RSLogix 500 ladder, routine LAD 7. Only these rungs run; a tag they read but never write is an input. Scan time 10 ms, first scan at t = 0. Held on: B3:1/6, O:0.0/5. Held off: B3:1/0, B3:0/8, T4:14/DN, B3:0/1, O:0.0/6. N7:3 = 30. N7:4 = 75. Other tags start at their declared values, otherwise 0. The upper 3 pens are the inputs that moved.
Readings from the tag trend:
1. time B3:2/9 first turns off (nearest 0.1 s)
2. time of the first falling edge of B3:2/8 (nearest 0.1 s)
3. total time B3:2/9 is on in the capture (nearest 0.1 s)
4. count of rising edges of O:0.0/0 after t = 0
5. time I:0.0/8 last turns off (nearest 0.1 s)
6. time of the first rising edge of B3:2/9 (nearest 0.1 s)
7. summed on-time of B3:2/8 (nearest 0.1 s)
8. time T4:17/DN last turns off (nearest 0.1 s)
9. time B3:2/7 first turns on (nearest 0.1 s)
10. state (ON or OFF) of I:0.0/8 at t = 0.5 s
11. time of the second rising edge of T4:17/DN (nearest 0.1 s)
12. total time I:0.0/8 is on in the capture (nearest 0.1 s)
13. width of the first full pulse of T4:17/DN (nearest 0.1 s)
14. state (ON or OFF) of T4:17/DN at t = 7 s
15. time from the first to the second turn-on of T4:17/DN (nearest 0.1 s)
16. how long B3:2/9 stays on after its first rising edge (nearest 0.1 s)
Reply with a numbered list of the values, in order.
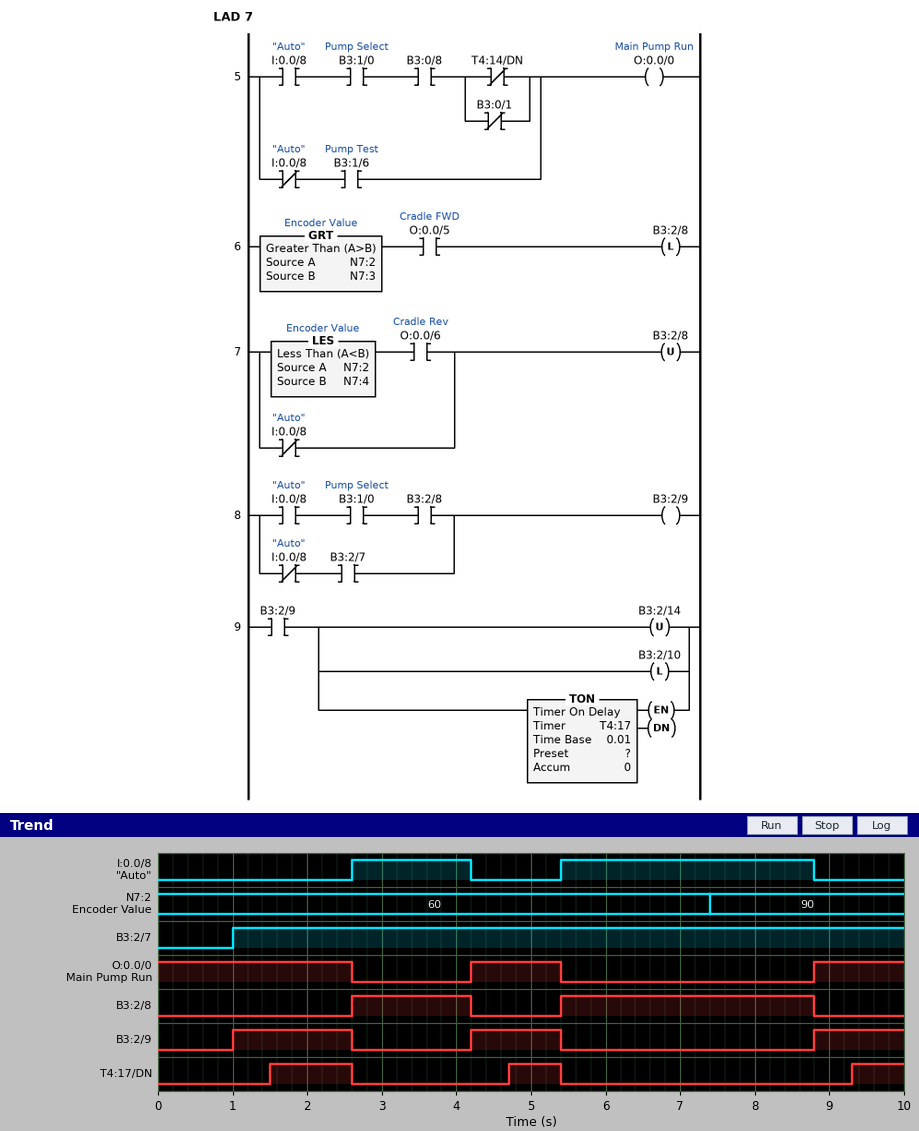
1. 2.6 s
2. 4.2 s
3. 4.0 s
4. 2
5. 8.8 s
6. 1.0 s
7. 5.0 s
8. 5.4 s
9. 1.0 s
10. OFF
11. 4.7 s
12. 5.0 s
13. 1.1 s
14. OFF
15. 3.2 s
16. 1.6 s
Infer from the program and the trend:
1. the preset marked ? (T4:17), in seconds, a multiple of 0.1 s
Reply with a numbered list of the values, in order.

1. 0.5 s
